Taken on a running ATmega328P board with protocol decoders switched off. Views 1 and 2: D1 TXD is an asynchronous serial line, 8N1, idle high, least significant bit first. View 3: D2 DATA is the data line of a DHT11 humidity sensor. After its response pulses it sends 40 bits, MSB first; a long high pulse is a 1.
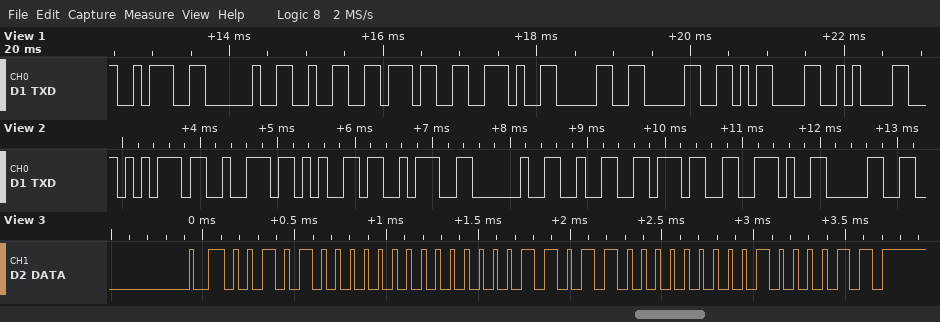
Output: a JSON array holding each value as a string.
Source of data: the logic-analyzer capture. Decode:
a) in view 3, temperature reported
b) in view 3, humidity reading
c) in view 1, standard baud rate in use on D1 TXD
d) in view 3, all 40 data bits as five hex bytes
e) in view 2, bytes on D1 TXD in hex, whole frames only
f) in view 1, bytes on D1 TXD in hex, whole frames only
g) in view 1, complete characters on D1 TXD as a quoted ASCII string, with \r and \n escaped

["27.0 °C", "40 %", "9600 baud", "28 00 1B 00 43", "75 72 65 3A 20 32 37 2E 30", "3A 20 32 37 2E 30 30 0D 0A", "\": 27.00\\r\\n\""]
